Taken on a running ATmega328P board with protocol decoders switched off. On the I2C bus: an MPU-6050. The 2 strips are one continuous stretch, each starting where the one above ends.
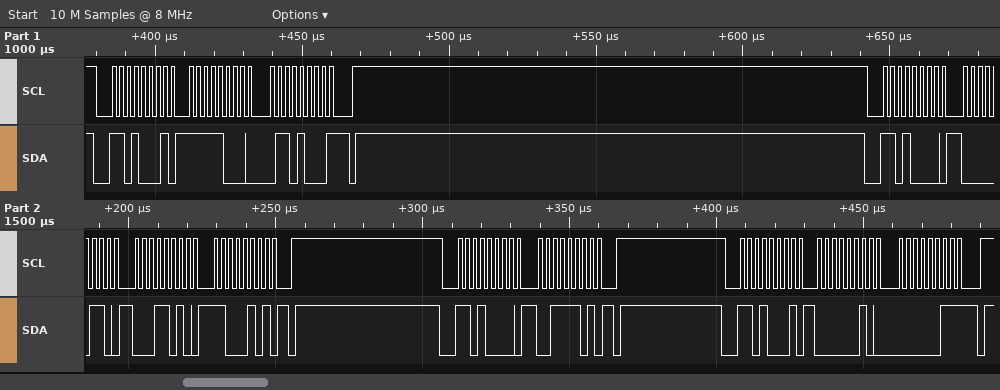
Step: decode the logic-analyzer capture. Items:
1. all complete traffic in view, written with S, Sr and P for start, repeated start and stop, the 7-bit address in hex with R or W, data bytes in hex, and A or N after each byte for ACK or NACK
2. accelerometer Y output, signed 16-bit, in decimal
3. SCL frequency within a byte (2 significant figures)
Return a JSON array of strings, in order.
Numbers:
["S 68R A F8 A 68 N P S 68W A 06 A 1A A C5 A P S 68W A 3D A P S 68R A 02 A 03 N P", "515", "400 kHz"]
